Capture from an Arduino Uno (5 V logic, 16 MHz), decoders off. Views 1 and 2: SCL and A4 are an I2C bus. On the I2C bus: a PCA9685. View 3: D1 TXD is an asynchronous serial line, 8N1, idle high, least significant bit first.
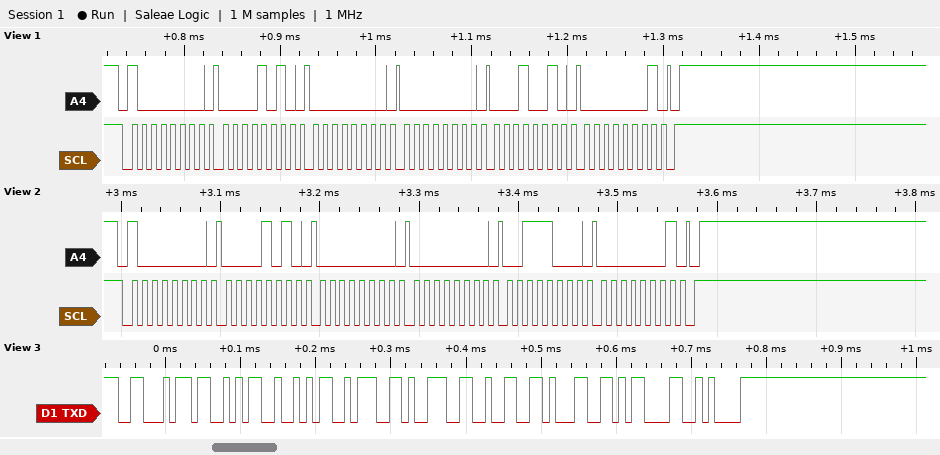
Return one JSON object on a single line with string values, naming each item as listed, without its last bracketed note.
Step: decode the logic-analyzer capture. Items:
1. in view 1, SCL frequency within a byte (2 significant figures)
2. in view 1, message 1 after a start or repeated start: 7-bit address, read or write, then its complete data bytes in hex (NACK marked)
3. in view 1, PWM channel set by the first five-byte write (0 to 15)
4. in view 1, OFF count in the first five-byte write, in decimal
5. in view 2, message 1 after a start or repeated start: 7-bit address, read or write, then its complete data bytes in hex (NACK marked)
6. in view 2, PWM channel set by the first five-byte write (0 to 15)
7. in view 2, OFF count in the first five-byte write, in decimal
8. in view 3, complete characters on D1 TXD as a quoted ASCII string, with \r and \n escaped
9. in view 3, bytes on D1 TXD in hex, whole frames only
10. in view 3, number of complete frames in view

{"in view 1, SCL frequency within a byte": "100 kHz", "in view 1, message 1 after a start or repeated start: 7-bit address, read or write, then its complete data bytes in hex": "0x40 write: 0A 00 00 12 01", "in view 1, PWM channel set by the first five-byte write": "1", "in view 1, OFF count in the first five-byte write, in decimal": "274", "in view 2, message 1 after a start or repeated start: 7-bit address, read or write, then its complete data bytes in hex": "0x40 write: 0A 00 00 38 01", "in view 2, PWM channel set by the first five-byte write": "1", "in view 2, OFF count in the first five-byte write, in decimal": "312", "in view 3, complete characters on D1 TXD as a quoted ASCII string, with \\r and \\n escaped": "\"FSR:921\\r\\n\"", "in view 3, bytes on D1 TXD in hex, whole frames only": "46 53 52 3A 39 32 31 0D 0A", "in view 3, number of complete frames in view": "9"}
